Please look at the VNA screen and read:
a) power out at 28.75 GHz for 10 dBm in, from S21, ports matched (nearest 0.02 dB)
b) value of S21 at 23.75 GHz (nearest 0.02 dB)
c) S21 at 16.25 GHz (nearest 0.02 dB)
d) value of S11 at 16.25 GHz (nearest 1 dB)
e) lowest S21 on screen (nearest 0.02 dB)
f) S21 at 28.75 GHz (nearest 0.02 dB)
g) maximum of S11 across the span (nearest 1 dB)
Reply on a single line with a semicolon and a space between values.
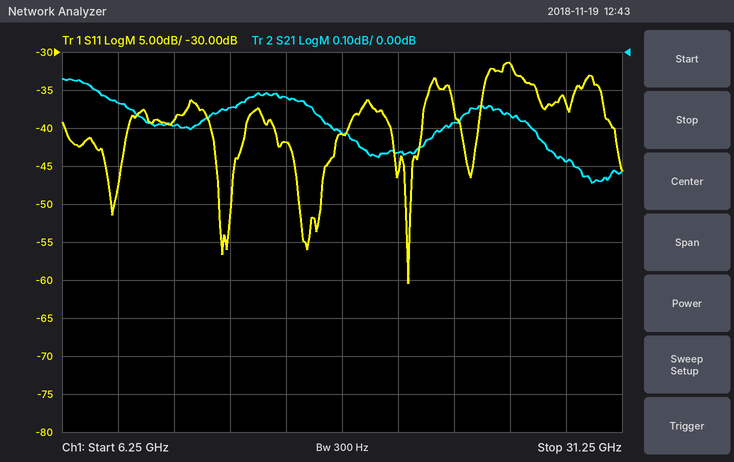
9.72 dBm; -0.18 dB; -0.12 dB; -42 dB; -0.34 dB; -0.28 dB; -31 dB
